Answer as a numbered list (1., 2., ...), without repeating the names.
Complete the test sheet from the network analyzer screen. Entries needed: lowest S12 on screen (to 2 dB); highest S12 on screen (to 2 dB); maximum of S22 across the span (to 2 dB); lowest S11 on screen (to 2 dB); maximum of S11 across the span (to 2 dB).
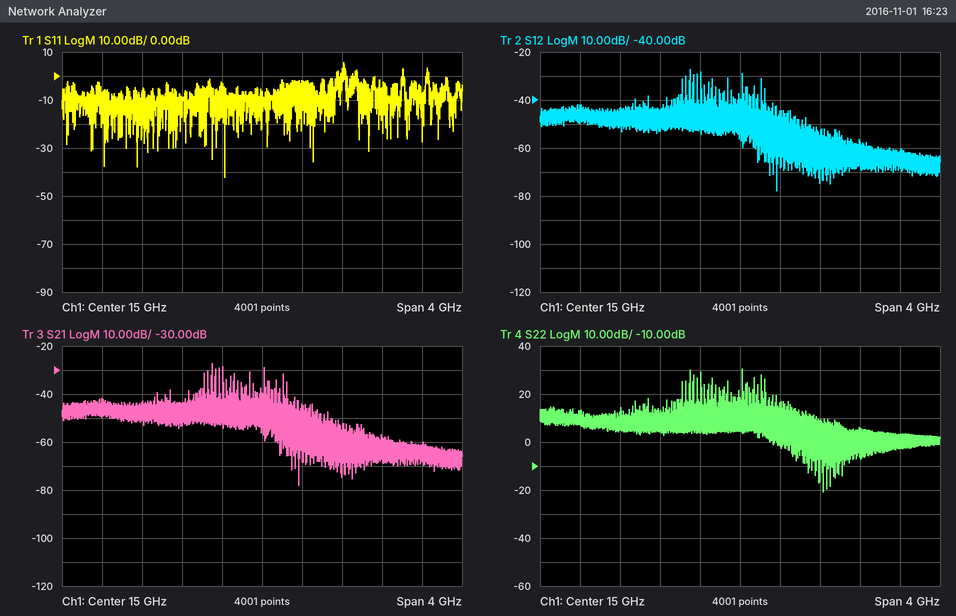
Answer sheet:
1. -78 dB
2. -28 dB
3. 30 dB
4. -42 dB
5. 6 dB
